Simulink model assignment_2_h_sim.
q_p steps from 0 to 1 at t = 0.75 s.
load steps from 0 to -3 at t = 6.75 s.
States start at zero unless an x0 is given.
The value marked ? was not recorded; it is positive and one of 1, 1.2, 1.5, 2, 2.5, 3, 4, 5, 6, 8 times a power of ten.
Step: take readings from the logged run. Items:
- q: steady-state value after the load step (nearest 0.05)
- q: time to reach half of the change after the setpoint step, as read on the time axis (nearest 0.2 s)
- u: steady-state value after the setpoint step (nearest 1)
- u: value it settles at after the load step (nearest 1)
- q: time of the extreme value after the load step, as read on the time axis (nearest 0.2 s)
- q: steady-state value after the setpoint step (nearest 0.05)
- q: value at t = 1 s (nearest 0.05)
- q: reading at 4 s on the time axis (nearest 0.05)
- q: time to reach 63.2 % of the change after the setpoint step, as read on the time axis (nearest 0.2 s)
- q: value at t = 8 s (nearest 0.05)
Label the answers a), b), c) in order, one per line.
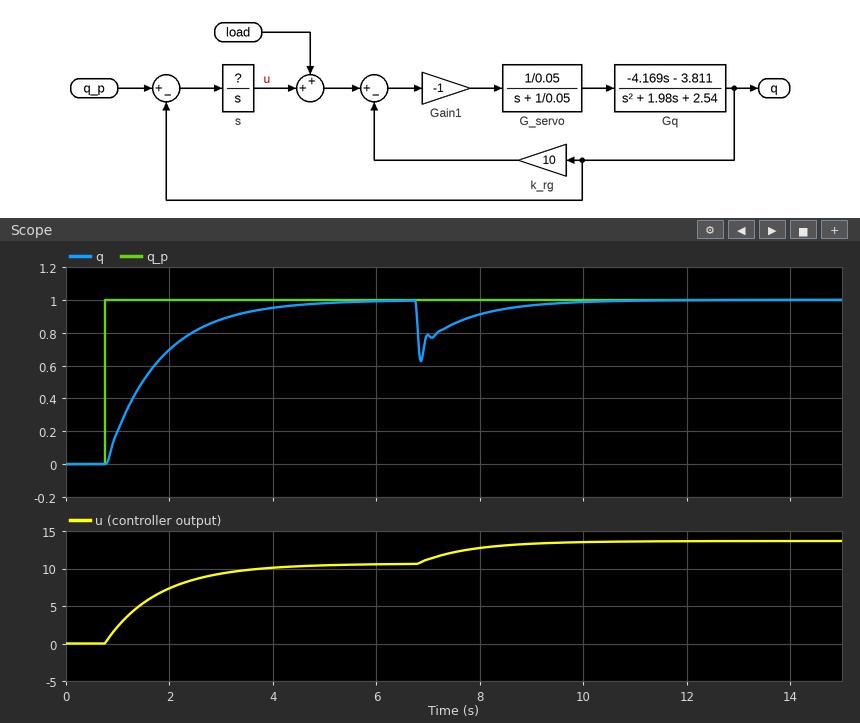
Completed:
a) 1.00
b) 1.4 s
c) 11
d) 14
e) 6.8 s
f) 1.00
g) 0.20
h) 0.95
i) 1.8 s
j) 0.90
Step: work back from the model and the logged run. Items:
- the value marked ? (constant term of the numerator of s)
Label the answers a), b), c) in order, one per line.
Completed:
a) 10
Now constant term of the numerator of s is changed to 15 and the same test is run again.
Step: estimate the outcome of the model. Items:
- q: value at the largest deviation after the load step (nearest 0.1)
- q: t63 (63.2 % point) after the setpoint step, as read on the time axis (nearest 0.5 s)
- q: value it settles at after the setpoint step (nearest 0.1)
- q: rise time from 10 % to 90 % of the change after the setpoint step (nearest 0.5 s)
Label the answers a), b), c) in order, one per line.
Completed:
a) 0.6
b) 1.5 s
c) 1.0
d) 1.5 s
